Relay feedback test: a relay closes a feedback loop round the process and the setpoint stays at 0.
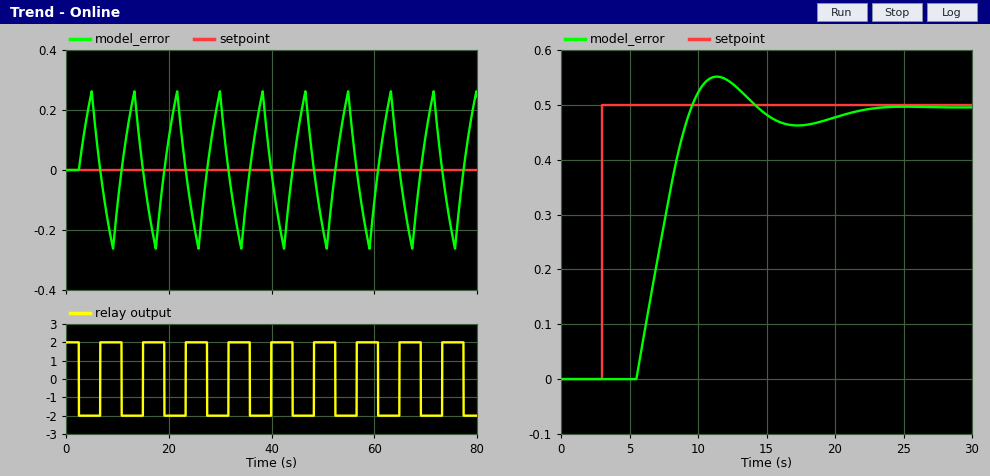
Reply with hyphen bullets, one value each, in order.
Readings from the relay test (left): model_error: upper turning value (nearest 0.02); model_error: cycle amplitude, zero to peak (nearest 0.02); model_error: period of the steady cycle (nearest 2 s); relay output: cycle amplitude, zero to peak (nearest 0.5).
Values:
- 0.26
- 0.26
- 8 s
- 2.0
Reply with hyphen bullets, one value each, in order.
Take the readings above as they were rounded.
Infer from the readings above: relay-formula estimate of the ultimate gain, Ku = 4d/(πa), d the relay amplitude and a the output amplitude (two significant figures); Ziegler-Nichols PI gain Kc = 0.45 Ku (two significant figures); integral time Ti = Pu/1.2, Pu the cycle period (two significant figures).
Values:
- 9.8
- 4.4
- 6.7 s
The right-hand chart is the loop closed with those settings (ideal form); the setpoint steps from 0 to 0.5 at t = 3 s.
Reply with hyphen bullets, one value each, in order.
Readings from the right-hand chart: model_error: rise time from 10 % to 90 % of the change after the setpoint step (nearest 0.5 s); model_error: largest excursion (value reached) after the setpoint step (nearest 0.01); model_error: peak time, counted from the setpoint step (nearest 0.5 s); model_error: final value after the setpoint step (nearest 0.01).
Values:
- 3.0 s
- 0.55
- 8.5 s
- 0.50
